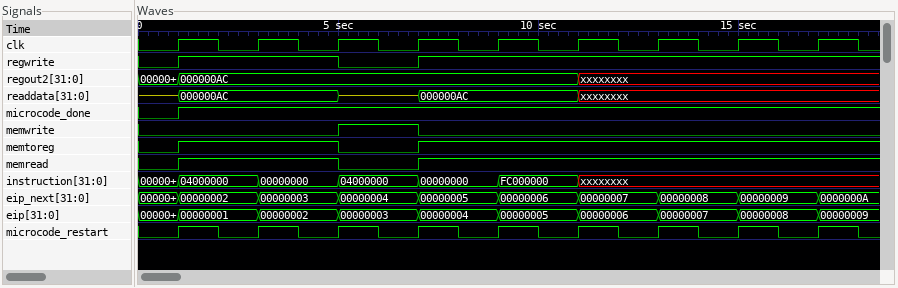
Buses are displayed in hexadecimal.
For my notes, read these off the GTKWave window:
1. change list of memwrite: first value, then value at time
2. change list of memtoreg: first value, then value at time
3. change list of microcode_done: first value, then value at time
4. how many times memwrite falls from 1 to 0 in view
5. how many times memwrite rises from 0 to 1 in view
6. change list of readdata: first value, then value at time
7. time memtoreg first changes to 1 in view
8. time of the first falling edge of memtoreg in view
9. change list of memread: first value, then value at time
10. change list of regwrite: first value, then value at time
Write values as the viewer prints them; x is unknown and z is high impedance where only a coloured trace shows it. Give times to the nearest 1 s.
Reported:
0, 1 at 5 s, 0 at 7 s
0, 1 at 1 s, 0 at 5 s, 1 at 7 s
0, 1 at 1 s
1
1
z, 000000AC at 1 s, z at 5 s, 000000AC at 7 s, xxxxxxxx at 11 s
1 s
5 s
0, 1 at 1 s, 0 at 5 s, 1 at 7 s
0, 1 at 1 s, 0 at 5 s, 1 at 7 s
